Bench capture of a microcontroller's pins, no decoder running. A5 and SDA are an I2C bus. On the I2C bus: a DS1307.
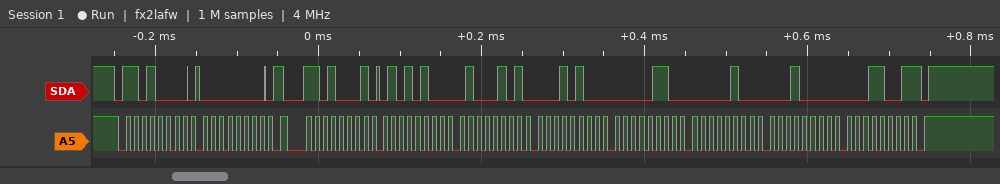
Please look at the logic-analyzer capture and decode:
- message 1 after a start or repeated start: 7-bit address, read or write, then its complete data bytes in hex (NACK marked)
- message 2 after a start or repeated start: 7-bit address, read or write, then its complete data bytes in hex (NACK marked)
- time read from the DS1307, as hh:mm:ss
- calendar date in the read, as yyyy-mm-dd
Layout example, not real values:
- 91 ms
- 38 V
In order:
- 0x68 write: 00
- 0x68 read: 54 45 14 06 04 10 19 NACK
- 14:45:54
- 2019-10-04
